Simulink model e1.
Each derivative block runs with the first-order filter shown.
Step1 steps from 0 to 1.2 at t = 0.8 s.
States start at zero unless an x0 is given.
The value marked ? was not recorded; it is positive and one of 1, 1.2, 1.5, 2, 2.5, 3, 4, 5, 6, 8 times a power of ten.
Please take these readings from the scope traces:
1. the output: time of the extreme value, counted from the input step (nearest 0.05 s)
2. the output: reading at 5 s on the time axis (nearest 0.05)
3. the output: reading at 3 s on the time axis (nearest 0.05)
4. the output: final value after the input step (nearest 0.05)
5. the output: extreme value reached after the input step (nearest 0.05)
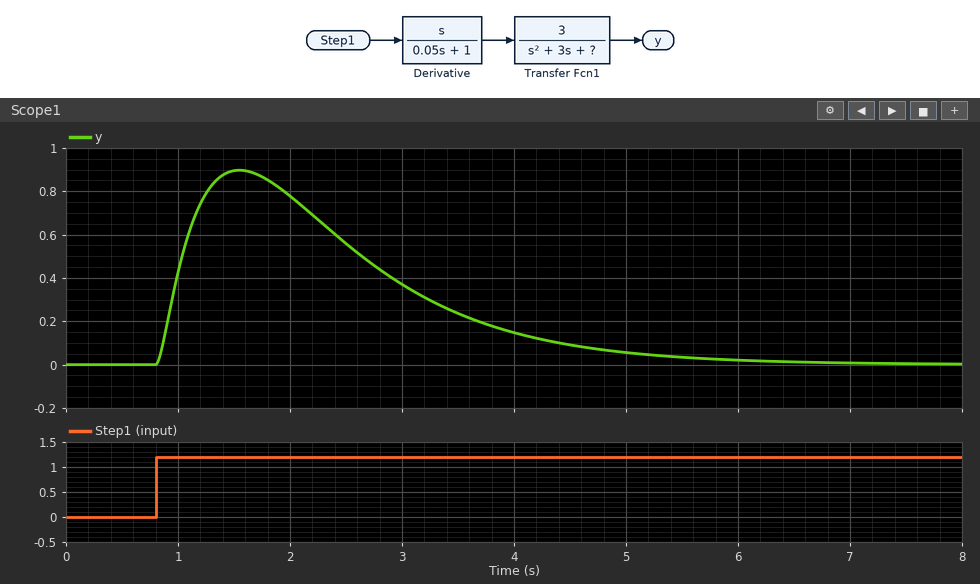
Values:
0.75 s
0.05
0.35
0.00
0.90
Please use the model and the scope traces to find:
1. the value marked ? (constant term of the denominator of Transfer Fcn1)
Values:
2
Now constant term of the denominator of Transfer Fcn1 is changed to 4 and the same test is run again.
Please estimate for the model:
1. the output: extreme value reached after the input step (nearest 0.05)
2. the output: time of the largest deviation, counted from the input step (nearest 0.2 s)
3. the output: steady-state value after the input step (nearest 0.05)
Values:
0.80
0.6 s
0.00
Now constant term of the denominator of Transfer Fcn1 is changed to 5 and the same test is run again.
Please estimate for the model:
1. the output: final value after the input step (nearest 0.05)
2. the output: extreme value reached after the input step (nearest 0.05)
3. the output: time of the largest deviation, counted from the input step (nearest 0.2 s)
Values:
0.00
0.75
0.6 s
